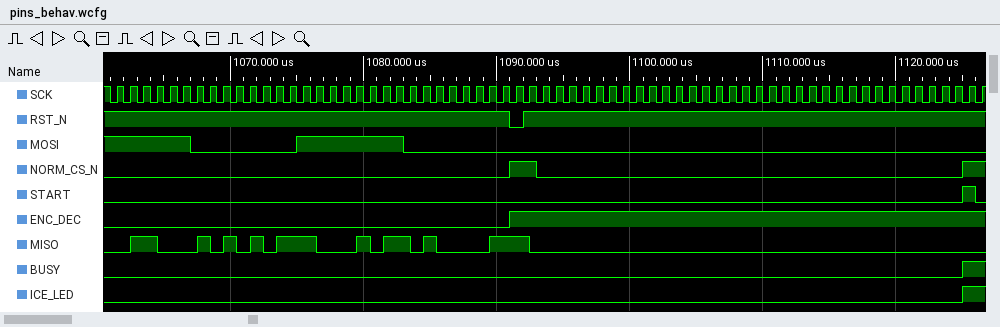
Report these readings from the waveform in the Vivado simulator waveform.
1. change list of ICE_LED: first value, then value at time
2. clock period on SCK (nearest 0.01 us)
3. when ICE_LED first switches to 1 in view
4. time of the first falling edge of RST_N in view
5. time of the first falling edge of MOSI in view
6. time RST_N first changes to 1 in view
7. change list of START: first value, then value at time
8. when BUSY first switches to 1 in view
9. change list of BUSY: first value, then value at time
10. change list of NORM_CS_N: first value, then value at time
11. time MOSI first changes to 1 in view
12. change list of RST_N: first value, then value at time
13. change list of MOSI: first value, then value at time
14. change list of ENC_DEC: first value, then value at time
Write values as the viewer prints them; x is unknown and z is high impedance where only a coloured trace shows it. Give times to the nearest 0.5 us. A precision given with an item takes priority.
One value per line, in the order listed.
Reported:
0, 1 at 1125 us
1 us
1125 us
1091 us
1067 us
1092 us
0, 1 at 1125 us, 0 at 1126 us
1125 us
0, 1 at 1125 us
0, 1 at 1091 us, 0 at 1093 us, 1 at 1125 us
1075 us
1, 0 at 1091 us, 1 at 1092 us
1, 0 at 1067 us, 1 at 1075 us, 0 at 1083 us
0, 1 at 1091 us
